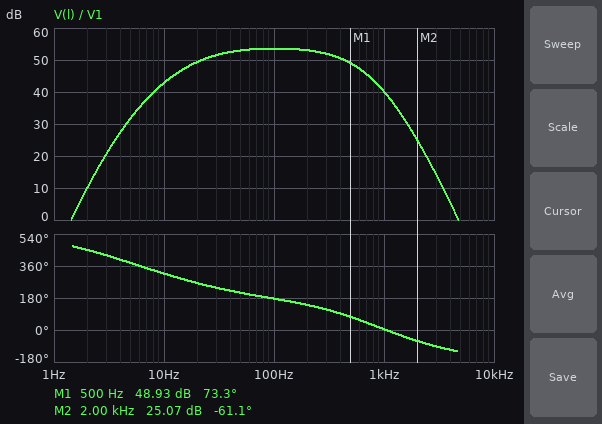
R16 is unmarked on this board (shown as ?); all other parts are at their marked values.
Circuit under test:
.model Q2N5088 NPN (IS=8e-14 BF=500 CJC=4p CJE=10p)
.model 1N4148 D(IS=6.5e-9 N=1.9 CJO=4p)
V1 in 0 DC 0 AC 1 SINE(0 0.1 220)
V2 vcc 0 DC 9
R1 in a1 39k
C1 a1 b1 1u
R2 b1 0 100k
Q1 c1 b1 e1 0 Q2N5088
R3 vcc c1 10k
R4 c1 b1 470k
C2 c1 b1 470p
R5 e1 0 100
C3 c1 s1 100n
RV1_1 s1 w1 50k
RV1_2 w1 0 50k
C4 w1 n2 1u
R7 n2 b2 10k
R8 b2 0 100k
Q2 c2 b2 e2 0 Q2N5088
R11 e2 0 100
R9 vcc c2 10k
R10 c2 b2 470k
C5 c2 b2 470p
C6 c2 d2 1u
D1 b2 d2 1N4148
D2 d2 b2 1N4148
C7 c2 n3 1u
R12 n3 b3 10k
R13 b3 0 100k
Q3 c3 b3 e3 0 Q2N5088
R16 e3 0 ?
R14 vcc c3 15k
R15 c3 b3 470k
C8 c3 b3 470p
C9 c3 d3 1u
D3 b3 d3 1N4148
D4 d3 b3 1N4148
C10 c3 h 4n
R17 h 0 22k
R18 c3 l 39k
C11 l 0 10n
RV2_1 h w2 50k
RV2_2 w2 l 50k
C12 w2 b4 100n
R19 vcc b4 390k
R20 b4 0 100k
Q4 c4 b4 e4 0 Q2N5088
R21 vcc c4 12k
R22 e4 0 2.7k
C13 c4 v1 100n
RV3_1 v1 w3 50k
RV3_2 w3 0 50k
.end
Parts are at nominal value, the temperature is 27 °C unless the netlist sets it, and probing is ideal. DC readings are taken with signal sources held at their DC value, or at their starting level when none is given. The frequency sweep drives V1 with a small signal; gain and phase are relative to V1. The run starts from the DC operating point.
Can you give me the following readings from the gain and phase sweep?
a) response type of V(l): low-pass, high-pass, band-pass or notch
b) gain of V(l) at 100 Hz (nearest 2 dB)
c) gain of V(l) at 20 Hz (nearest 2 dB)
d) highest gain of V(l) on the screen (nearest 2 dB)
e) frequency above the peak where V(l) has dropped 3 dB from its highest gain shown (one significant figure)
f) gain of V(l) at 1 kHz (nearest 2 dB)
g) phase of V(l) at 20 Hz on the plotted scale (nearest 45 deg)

band-pass
54 dB
50 dB
54 dB
400 Hz
40 dB
270 deg
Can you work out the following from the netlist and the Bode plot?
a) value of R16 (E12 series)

120 Ω
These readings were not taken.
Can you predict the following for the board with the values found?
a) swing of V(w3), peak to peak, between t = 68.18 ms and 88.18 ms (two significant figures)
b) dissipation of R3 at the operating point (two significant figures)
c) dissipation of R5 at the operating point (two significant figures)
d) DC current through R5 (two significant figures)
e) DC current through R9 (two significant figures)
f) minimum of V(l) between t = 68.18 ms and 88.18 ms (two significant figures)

450 mV
2.4 mW
24 µW
490 µA
490 µA
2.6 V
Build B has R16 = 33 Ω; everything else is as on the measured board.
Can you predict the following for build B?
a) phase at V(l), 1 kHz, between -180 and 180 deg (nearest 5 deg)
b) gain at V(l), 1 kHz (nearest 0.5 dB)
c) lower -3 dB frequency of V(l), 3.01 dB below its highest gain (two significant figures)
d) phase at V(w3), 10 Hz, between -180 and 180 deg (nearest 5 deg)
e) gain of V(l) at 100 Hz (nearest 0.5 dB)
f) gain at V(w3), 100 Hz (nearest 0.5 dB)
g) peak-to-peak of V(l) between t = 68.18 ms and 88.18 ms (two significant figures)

0 deg
41.5 dB
25 Hz
-105 deg
55.0 dB
53.0 dB
590 mV
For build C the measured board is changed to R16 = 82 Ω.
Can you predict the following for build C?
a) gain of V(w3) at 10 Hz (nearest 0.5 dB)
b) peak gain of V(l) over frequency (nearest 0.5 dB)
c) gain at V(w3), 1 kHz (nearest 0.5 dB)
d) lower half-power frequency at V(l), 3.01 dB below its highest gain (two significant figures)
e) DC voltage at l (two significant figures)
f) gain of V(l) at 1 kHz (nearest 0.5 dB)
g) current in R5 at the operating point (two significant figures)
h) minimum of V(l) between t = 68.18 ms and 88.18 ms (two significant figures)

31.5 dB
54.0 dB
38.5 dB
25 Hz
2.8 V
40.5 dB
490 µA
2.5 V
